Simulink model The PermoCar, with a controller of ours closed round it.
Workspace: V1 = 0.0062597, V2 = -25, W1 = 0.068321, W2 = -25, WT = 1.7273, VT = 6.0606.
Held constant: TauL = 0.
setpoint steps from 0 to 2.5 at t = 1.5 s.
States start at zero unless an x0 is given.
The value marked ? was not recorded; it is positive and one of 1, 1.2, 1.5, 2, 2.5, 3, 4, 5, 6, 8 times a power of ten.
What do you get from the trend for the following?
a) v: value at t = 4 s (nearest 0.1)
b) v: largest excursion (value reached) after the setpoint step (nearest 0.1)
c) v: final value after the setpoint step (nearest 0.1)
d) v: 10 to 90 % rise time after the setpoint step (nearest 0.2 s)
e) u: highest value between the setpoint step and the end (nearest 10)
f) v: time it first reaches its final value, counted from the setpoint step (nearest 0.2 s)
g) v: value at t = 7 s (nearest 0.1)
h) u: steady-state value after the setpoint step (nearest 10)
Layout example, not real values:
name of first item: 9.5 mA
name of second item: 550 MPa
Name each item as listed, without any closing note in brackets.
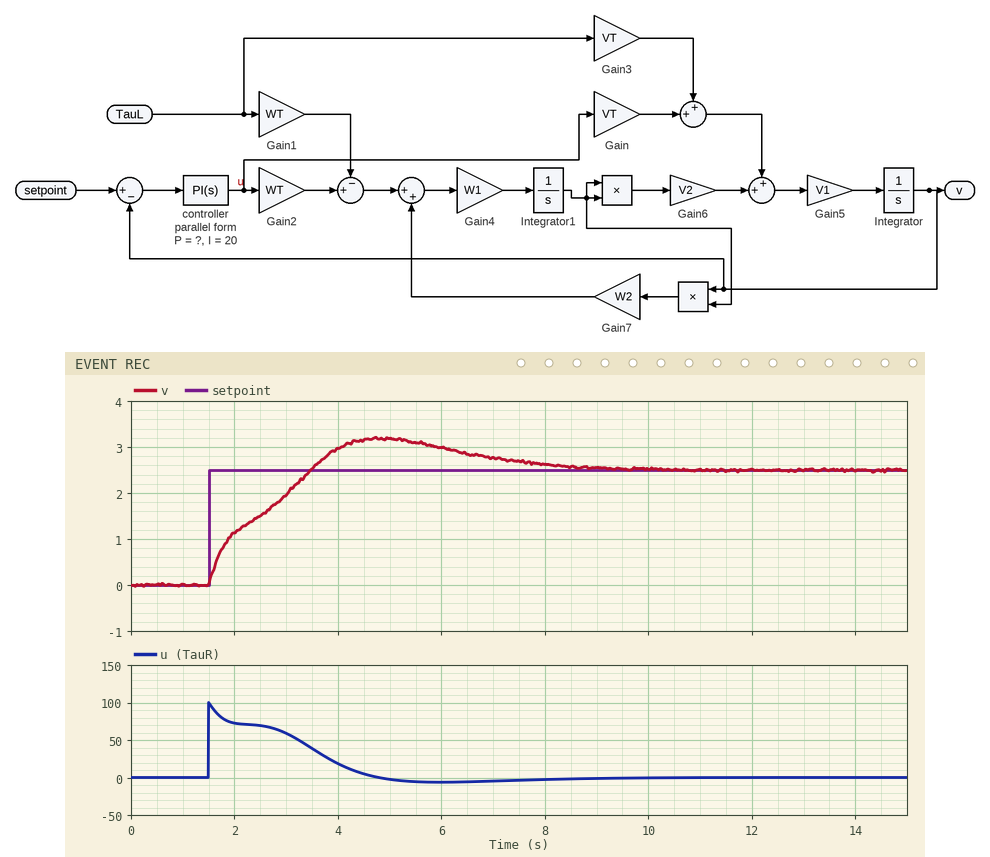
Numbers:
v: value at t = 4 s: 3.0
v: largest excursion (value reached) after the setpoint step: 3.2
v: final value after the setpoint step: 2.5
v: 10 to 90 % rise time after the setpoint step: 1.6 s
u: highest value between the setpoint step and the end: 100
v: time it first reaches its final value, counted from the setpoint step: 2.0 s
v: value at t = 7 s: 2.8
u: steady-state value after the setpoint step: 0
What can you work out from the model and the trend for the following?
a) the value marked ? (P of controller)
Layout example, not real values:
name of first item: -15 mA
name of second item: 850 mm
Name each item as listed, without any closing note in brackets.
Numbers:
the value marked ?: 40
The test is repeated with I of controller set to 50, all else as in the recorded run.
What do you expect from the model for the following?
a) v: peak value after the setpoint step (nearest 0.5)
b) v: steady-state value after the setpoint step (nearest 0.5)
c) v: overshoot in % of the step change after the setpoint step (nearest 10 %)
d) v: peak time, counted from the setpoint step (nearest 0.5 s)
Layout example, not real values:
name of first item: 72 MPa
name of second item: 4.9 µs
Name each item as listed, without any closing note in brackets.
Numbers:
v: peak value after the setpoint step: 3.5
v: steady-state value after the setpoint step: 2.5
v: overshoot in % of the step change after the setpoint step: 40 %
v: peak time, counted from the setpoint step: 2.5 s
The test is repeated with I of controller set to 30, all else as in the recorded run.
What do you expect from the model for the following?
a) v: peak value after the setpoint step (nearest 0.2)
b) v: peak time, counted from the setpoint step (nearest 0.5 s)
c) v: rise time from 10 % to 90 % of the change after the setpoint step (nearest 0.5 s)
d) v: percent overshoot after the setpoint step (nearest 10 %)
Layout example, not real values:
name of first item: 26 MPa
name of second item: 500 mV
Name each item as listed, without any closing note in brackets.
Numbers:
v: peak value after the setpoint step: 3.4
v: peak time, counted from the setpoint step: 3.0 s
v: rise time from 10 % to 90 % of the change after the setpoint step: 1.5 s
v: percent overshoot after the setpoint step: 30 %
